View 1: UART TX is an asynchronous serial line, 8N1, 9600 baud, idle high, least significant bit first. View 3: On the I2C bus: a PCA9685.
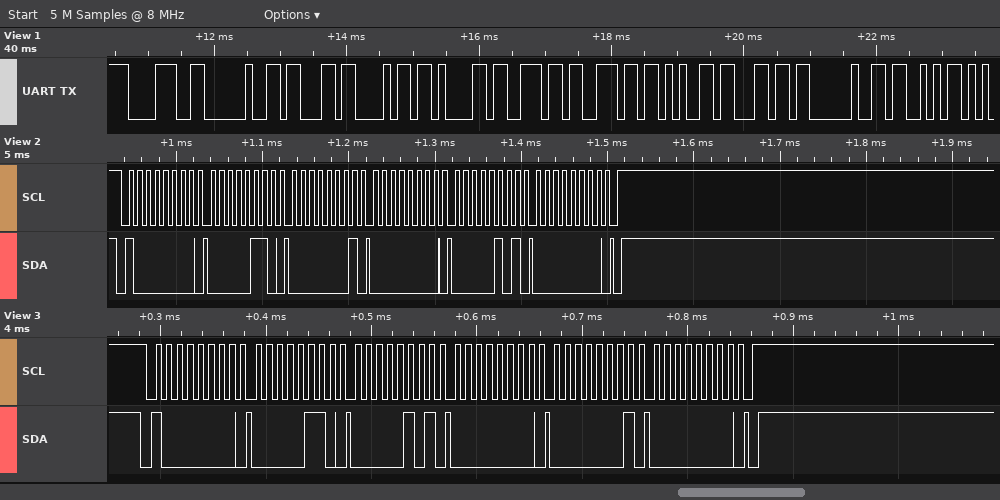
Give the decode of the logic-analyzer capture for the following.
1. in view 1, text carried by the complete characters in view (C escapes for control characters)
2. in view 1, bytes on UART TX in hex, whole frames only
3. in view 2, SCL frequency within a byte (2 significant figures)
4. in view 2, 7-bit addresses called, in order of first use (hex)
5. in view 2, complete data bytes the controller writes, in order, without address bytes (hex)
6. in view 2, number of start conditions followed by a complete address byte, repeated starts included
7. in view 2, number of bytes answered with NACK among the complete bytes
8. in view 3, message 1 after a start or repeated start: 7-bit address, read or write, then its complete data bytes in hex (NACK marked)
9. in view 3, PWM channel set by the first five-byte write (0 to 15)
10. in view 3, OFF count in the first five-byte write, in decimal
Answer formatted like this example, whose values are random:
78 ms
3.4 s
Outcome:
"8 channel S"
38 20 63 68 61 6E 6E 65 6C 20 53
100 kHz
0x40
06 01 00 05 00
1
0
0x40 write: 06 05 00 01 00
0
1
